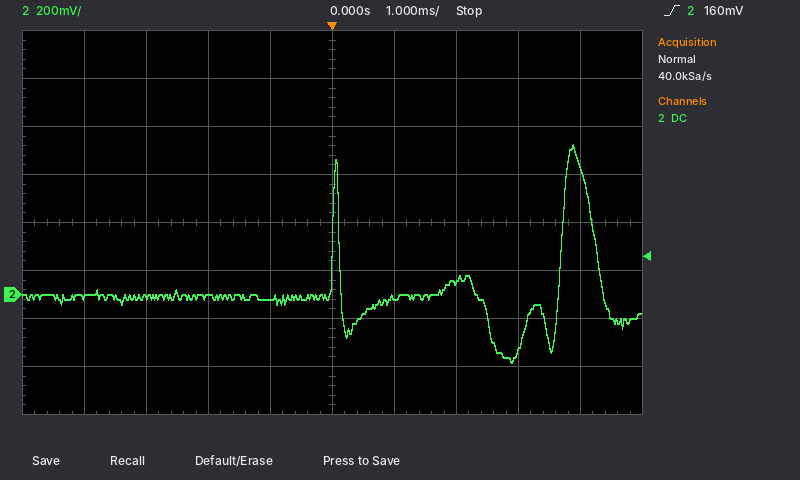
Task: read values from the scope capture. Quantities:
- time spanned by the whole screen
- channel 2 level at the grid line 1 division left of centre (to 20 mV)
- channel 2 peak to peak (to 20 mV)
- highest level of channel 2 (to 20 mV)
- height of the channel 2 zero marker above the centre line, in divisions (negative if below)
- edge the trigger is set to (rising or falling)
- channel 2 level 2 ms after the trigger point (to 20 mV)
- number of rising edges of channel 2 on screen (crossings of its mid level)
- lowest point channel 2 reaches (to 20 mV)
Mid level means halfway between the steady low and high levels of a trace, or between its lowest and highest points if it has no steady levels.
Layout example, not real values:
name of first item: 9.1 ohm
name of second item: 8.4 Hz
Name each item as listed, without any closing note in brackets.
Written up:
time spanned by the whole screen: 10 ms
channel 2 level at the grid line 1 division left of centre: -20 mV
channel 2 peak to peak: 900 mV
highest level of channel 2: 620 mV
height of the channel 2 zero marker above the centre line, in divisions: -1.5 div
edge the trigger is set to: rising
channel 2 level 2 ms after the trigger point: 60 mV
number of rising edges of channel 2 on screen: 2
lowest point channel 2 reaches: -280 mV
